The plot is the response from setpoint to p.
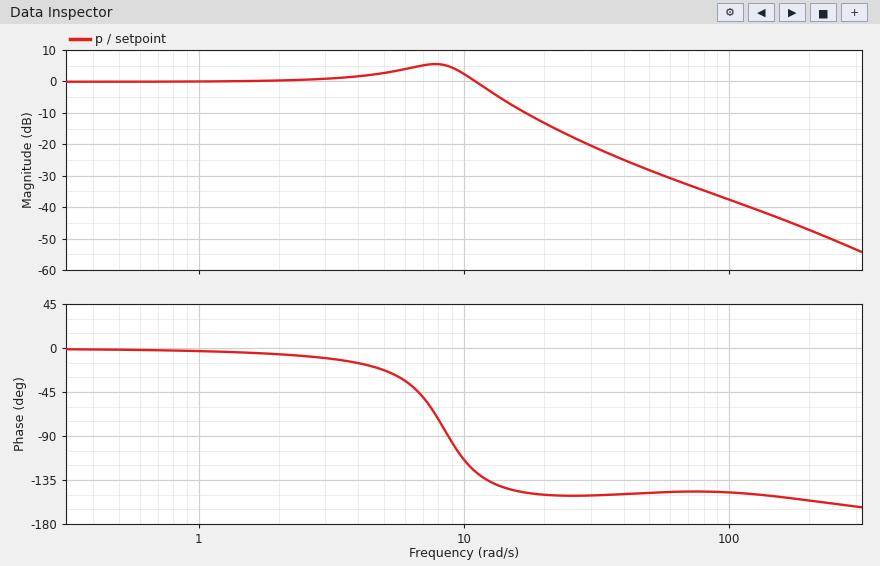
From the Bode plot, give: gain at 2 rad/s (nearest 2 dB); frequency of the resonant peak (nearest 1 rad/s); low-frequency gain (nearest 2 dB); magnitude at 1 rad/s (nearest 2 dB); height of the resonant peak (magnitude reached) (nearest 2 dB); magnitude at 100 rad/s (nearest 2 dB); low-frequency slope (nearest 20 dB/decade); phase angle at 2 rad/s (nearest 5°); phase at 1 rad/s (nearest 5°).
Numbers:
0 dB
8 rad/s
0 dB
0 dB
6 dB
-38 dB
0 dB/decade
-5°
-5°
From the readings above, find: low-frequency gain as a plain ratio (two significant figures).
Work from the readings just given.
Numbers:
1.0
